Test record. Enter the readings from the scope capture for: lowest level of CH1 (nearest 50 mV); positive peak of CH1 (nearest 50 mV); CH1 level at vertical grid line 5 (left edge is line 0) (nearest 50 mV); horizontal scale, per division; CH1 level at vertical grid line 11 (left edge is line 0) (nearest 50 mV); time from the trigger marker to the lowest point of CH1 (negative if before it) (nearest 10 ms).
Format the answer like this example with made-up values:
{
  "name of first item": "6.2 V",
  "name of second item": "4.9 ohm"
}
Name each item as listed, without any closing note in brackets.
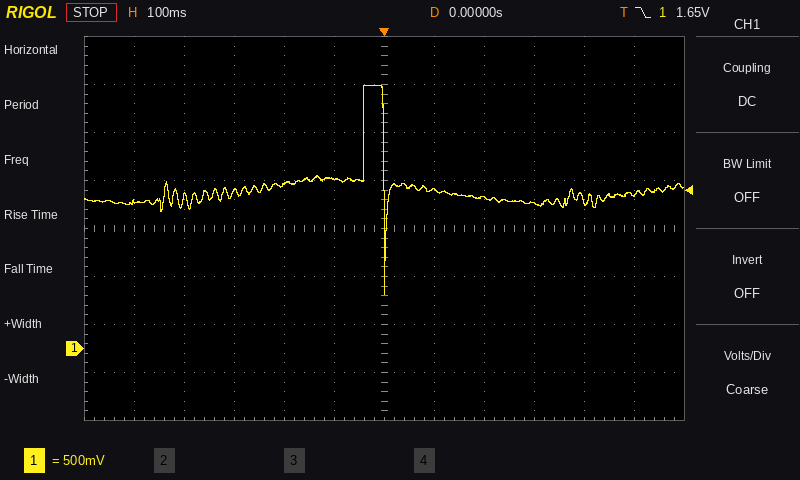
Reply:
{
  "lowest level of CH1": "550 mV",
  "positive peak of CH1": "2.75 V",
  "CH1 level at vertical grid line 5 (left edge is line 0)": "1.75 V",
  "horizontal scale, per division": "100 ms",
  "CH1 level at vertical grid line 11 (left edge is line 0)": "1.60 V",
  "time from the trigger marker to the lowest point of CH1 (negative if before it)": "0 ms"
}
